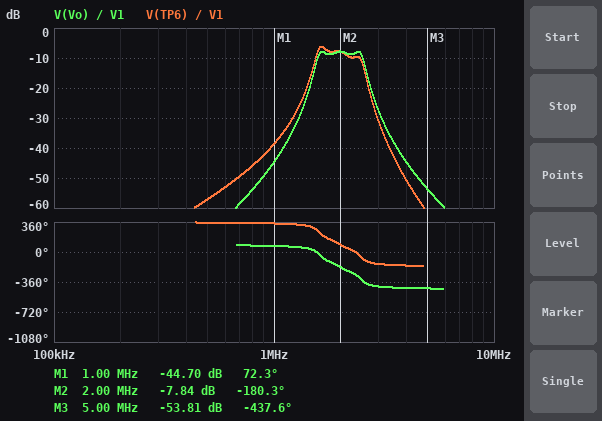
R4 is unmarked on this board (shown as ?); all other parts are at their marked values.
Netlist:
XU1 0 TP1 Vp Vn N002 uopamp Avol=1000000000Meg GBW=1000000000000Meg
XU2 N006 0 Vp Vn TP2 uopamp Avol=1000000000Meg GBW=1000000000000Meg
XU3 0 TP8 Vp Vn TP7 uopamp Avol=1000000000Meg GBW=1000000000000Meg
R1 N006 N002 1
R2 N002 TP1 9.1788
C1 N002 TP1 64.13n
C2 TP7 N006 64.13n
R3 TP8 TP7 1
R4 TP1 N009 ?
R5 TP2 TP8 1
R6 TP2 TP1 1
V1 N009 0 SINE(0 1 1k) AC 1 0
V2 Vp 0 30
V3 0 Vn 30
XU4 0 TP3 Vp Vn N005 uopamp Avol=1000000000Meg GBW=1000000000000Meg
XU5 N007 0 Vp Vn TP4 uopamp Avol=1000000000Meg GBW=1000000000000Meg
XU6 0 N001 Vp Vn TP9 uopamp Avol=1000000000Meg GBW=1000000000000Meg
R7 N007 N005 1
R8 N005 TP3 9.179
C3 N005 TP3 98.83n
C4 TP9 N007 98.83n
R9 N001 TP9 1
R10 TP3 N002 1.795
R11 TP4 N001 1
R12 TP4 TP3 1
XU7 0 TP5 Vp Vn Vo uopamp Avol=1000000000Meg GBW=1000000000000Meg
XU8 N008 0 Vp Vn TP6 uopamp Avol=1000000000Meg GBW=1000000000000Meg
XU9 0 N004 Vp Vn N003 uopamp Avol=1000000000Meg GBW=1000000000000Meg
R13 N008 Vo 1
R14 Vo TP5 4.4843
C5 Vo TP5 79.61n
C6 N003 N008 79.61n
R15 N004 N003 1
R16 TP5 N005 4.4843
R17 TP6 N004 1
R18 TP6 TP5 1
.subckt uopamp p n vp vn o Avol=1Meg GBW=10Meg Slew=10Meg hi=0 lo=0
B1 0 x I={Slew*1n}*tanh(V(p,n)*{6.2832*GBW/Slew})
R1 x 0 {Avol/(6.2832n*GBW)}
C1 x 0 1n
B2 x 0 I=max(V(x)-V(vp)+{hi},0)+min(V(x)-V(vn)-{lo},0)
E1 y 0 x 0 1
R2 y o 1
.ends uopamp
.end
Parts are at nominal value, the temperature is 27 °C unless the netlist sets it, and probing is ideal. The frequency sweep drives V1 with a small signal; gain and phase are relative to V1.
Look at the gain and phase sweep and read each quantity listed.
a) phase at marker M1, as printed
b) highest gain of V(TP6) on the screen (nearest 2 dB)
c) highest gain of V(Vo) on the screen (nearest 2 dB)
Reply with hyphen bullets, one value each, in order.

- 72.3 deg
- -6 dB
- -8 dB
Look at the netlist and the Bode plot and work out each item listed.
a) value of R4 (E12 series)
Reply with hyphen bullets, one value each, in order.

- 6.8 Ω
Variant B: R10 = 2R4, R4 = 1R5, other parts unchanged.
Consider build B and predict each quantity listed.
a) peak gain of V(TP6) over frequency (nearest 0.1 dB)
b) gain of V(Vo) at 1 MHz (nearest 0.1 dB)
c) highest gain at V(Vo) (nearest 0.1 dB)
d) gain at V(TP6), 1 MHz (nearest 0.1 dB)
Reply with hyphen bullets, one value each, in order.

- 4.5 dB
- -34.1 dB
- 2.8 dB
- -28.1 dB
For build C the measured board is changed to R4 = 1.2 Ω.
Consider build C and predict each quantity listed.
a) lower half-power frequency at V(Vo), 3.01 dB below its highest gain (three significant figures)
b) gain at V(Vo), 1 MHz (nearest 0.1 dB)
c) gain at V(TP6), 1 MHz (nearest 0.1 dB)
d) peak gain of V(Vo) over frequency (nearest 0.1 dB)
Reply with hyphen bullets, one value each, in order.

- 1.57 MHz
- -29.6 dB
- -23.6 dB
- 7.2 dB
